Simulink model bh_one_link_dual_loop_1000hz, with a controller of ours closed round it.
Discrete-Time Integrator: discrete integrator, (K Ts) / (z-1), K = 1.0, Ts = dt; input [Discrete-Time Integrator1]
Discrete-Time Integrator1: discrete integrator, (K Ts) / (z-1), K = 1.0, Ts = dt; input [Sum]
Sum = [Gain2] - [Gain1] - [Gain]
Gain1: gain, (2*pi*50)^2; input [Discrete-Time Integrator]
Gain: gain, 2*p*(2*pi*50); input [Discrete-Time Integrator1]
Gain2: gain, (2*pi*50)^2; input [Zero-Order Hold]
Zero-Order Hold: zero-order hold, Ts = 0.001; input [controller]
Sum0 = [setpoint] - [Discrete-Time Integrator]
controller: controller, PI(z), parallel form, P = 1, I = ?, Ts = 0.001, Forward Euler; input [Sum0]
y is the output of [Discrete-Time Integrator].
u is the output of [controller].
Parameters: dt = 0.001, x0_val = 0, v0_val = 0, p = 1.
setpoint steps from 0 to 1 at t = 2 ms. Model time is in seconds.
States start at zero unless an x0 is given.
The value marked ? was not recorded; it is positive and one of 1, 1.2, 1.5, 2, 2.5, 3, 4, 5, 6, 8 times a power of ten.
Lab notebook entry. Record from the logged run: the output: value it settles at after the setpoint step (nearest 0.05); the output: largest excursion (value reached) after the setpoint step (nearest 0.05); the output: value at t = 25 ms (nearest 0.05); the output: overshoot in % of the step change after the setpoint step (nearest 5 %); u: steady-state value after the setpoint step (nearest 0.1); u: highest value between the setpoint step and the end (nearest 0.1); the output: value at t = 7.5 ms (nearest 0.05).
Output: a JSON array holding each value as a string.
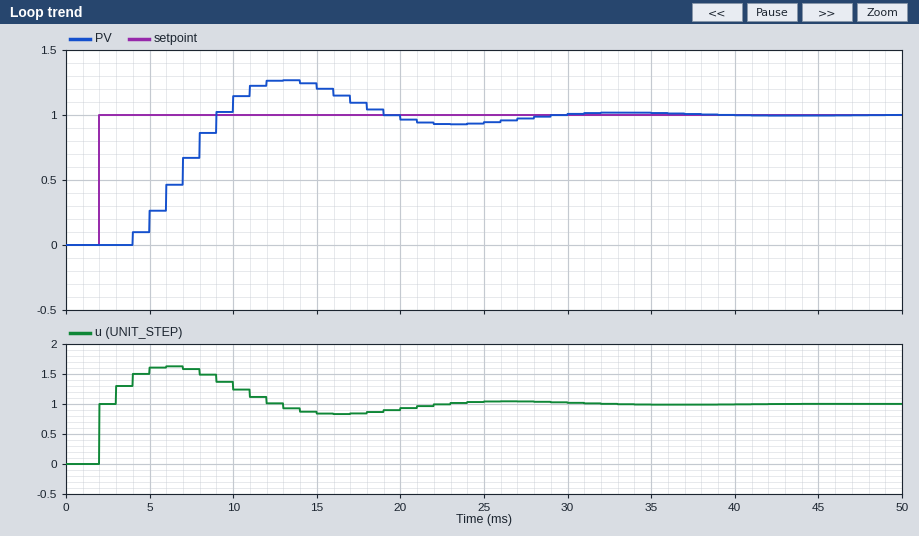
["1.00", "1.25", "0.95", "25 %", "1.0", "1.6", "0.65"]
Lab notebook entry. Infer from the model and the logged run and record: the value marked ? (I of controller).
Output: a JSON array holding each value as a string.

["300"]
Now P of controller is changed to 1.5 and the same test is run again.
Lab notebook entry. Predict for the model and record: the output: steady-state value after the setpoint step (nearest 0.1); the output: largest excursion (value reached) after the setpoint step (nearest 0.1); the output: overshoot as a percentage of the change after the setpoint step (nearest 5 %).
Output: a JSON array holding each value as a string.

["1.0", "1.2", "20 %"]
